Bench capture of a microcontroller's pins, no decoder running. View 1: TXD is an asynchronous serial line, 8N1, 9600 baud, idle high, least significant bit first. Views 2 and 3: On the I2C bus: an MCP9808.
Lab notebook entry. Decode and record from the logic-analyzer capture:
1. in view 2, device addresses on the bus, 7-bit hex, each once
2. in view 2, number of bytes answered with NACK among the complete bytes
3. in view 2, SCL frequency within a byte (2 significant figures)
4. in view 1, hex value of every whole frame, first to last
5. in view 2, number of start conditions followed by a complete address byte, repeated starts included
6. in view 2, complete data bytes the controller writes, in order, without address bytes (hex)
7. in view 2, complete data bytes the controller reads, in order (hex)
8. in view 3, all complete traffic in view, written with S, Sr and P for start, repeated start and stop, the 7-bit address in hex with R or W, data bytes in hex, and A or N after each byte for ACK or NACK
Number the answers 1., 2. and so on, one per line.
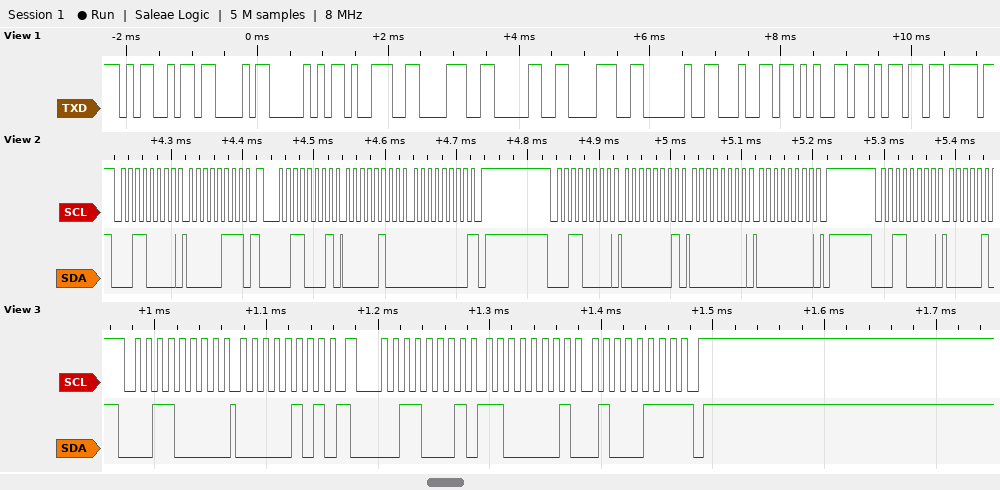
1. 0x18
2. 1
3. 100 kHz
4. 4D 43 50 39 38 30 38 20 64 65 6D
5. 4
6. 07 01 00 00
7. 04 00
8. S 18W A 05 A Sr 18R A C1 A 47 N P
